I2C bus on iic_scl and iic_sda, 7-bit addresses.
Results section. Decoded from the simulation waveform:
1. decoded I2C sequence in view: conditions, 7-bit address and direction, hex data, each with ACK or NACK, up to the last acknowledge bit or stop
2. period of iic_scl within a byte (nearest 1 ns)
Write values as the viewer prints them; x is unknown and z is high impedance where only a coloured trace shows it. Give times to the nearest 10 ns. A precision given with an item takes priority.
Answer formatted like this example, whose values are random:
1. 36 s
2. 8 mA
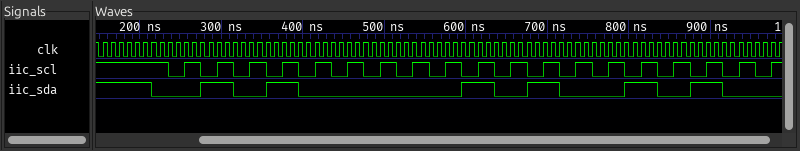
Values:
1. start, address 28 write ACK, A5 ACK
2. 40 ns
